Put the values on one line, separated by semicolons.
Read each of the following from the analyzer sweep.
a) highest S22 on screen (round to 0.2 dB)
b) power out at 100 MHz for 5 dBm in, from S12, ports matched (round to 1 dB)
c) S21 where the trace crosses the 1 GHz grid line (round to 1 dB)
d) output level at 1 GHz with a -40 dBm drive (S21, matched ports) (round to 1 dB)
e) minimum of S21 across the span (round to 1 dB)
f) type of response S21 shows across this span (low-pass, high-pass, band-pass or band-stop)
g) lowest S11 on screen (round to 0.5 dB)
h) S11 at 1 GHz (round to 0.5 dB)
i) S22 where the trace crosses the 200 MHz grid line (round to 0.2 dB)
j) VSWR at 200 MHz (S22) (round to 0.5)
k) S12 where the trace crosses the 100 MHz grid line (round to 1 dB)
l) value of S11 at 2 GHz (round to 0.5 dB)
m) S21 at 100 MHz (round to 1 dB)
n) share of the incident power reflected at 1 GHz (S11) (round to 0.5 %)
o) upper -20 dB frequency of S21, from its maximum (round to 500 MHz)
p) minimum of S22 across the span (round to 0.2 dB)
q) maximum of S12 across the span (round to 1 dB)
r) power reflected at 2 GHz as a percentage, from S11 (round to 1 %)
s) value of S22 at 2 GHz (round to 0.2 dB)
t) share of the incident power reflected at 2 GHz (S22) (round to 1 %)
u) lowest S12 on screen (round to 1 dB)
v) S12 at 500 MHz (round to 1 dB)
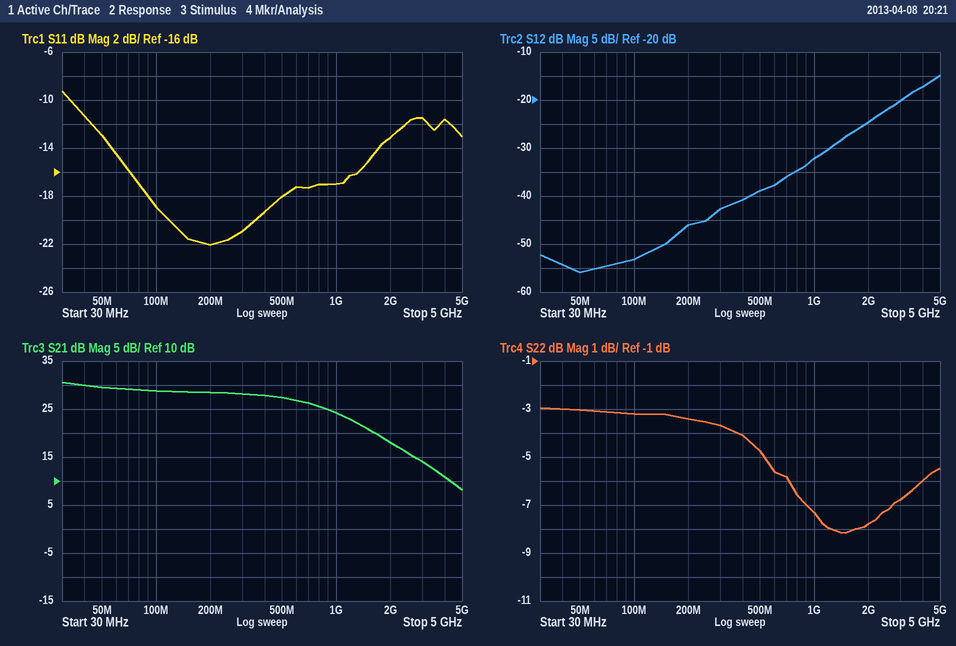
-3.0 dB; -48 dBm; 24 dB; -16 dBm; 8 dB; low-pass; -22.0 dB; -17.0 dB; -3.4 dB; 5.0; -53 dB; -13.0 dB; 29 dB; 2.0 %; 4.0 GHz; -8.2 dB; -15 dB; 5 %; -7.8 dB; 17 %; -56 dB; -39 dB
